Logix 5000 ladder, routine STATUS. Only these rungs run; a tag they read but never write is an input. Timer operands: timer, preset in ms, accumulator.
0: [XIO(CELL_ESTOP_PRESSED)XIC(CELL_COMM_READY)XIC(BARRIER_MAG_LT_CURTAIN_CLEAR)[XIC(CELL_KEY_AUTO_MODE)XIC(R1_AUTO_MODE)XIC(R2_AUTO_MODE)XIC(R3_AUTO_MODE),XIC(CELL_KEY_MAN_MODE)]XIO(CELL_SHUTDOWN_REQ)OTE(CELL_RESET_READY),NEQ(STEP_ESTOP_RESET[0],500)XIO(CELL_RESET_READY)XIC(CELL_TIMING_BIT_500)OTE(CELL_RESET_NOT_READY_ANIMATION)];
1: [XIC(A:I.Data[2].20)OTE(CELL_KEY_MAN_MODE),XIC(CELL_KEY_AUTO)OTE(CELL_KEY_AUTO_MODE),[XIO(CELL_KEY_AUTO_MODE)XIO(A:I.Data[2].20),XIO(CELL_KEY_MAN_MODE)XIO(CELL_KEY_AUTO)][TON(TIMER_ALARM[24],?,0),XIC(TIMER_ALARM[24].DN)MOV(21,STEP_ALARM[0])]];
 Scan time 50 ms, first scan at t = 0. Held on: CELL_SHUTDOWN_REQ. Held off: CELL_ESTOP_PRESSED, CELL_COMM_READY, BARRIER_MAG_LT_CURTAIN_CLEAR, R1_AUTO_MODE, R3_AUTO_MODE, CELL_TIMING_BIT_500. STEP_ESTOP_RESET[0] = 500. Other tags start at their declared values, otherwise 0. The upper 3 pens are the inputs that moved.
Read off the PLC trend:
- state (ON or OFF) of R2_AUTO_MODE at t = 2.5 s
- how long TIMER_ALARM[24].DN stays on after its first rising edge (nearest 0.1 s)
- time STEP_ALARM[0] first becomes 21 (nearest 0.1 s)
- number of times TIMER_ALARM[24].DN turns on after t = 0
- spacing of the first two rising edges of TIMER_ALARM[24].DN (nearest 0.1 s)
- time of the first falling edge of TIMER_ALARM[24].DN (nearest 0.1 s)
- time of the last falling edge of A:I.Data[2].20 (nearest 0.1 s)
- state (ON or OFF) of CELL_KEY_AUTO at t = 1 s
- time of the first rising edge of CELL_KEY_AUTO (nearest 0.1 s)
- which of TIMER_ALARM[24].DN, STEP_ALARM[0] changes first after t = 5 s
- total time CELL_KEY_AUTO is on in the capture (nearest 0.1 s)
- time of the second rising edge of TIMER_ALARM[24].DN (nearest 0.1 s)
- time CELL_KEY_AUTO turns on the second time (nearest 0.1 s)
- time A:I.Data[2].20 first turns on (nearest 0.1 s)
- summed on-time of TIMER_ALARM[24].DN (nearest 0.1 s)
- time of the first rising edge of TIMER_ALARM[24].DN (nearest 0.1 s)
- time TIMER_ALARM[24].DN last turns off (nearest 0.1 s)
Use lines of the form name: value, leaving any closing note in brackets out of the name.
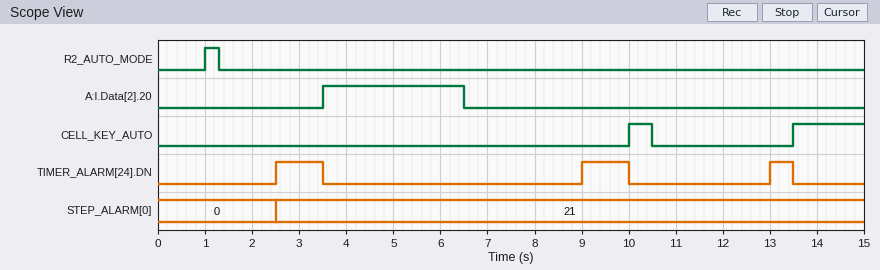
state (ON or OFF) of R2_AUTO_MODE at t = 2.5 s: OFF
how long TIMER_ALARM[24].DN stays on after its first rising edge: 1.0 s
time STEP_ALARM[0] first becomes 21: 2.5 s
number of times TIMER_ALARM[24].DN turns on after t = 0: 3
spacing of the first two rising edges of TIMER_ALARM[24].DN: 6.5 s
time of the first falling edge of TIMER_ALARM[24].DN: 3.5 s
time of the last falling edge of A:I.Data[2].20: 6.5 s
state (ON or OFF) of CELL_KEY_AUTO at t = 1 s: OFF
time of the first rising edge of CELL_KEY_AUTO: 10.0 s
which of TIMER_ALARM[24].DN, STEP_ALARM[0] changes first after t = 5 s: TIMER_ALARM[24].DN
total time CELL_KEY_AUTO is on in the capture: 2.0 s
time of the second rising edge of TIMER_ALARM[24].DN: 9.0 s
time CELL_KEY_AUTO turns on the second time: 13.5 s
time A:I.Data[2].20 first turns on: 3.5 s
summed on-time of TIMER_ALARM[24].DN: 2.5 s
time of the first rising edge of TIMER_ALARM[24].DN: 2.5 s
time TIMER_ALARM[24].DN last turns off: 13.5 s
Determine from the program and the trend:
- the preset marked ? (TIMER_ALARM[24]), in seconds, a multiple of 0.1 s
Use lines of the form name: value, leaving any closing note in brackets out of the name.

the preset marked ? (TIMER_ALARM[24]), in seconds, a multiple of 0.1 s: 2.5 s
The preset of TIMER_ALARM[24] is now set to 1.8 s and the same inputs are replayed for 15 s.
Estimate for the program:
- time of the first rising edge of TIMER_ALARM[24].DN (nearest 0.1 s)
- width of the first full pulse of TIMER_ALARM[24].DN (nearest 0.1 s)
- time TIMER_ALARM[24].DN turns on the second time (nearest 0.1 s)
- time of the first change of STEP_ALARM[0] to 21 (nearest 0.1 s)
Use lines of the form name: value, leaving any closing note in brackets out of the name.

time of the first rising edge of TIMER_ALARM[24].DN: 1.8 s
width of the first full pulse of TIMER_ALARM[24].DN: 1.7 s
time TIMER_ALARM[24].DN turns on the second time: 8.3 s
time of the first change of STEP_ALARM[0] to 21: 1.8 s
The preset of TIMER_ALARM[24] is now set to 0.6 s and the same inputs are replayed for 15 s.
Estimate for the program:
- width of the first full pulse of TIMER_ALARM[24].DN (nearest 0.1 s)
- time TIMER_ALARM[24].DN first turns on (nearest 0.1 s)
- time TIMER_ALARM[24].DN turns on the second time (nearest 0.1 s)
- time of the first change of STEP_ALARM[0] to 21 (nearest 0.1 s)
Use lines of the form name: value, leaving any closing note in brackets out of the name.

width of the first full pulse of TIMER_ALARM[24].DN: 2.9 s
time TIMER_ALARM[24].DN first turns on: 0.6 s
time TIMER_ALARM[24].DN turns on the second time: 7.1 s
time of the first change of STEP_ALARM[0] to 21: 0.6 s
